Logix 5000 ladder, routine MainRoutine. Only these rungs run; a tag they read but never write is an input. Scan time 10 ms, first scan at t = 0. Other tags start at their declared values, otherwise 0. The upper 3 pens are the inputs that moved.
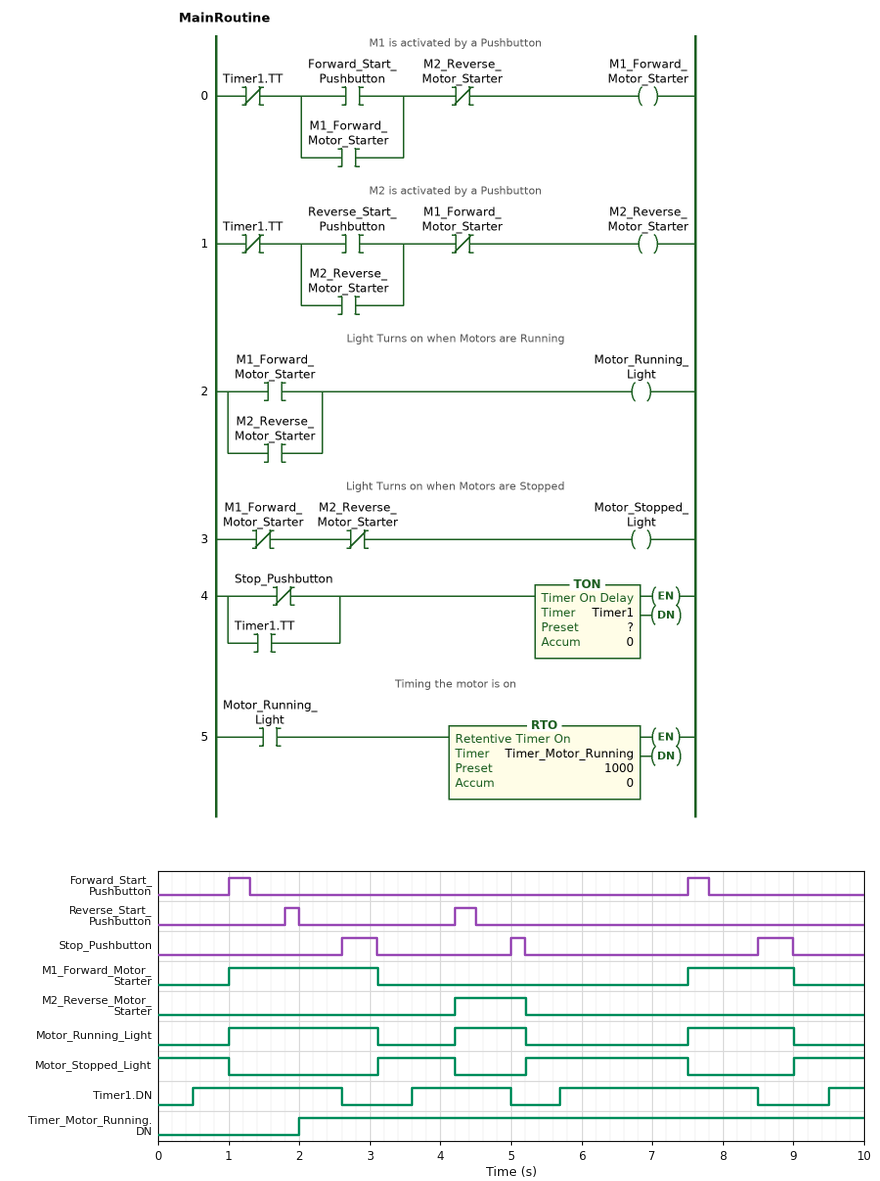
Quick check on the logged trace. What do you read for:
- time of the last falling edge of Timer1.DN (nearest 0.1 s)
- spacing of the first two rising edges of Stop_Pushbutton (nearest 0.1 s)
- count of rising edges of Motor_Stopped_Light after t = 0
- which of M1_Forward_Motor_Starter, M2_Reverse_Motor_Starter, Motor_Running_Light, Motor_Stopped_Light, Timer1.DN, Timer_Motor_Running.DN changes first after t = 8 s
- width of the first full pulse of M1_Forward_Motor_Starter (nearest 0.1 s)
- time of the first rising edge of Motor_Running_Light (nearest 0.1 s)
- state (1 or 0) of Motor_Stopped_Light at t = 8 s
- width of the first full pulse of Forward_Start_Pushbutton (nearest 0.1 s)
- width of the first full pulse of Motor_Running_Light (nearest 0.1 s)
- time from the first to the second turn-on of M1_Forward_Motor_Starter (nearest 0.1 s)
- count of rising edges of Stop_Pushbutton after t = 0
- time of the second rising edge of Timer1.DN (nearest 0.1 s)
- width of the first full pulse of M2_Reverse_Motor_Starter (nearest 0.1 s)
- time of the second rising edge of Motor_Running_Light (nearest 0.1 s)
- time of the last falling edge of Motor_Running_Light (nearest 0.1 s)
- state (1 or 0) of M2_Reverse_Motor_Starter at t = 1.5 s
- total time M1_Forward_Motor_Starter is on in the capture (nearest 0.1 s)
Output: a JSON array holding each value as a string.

["8.5 s", "2.4 s", "3", "Timer1.DN", "2.1 s", "1.0 s", "0", "0.3 s", "2.1 s", "6.5 s", "3", "3.6 s", "1.0 s", "4.2 s", "9.0 s", "0", "3.6 s"]
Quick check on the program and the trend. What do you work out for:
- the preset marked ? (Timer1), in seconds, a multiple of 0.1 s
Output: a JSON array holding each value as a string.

["0.5 s"]
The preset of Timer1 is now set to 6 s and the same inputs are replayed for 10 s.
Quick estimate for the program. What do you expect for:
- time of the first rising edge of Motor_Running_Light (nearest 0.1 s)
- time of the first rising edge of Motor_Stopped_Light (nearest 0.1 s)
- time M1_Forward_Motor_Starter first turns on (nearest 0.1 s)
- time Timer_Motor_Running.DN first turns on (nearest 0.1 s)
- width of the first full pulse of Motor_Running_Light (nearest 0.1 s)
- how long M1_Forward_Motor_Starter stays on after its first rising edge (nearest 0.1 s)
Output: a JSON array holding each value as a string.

["7.5 s", "9.0 s", "7.5 s", "8.5 s", "1.5 s", "1.5 s"]
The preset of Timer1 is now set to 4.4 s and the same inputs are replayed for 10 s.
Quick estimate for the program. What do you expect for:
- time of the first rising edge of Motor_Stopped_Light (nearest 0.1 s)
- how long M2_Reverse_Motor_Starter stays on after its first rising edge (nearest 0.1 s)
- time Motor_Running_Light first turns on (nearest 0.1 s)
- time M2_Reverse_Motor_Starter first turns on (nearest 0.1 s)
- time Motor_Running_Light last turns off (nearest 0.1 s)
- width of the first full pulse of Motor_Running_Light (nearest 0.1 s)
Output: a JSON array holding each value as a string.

["5.2 s", "0.8 s", "4.4 s", "4.4 s", "5.2 s", "0.8 s"]
